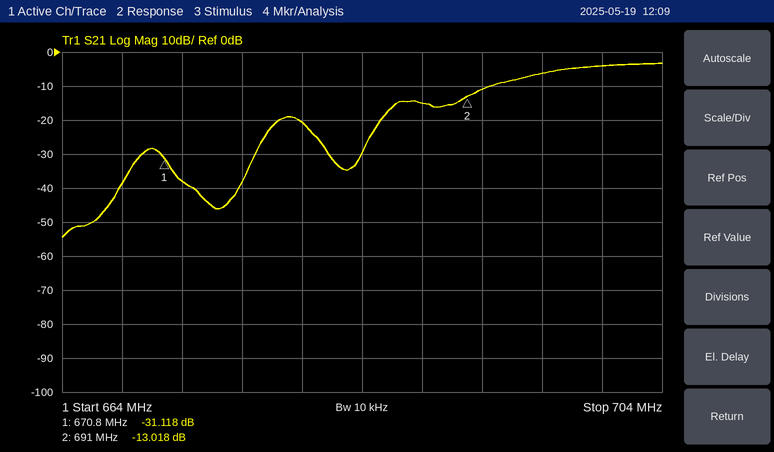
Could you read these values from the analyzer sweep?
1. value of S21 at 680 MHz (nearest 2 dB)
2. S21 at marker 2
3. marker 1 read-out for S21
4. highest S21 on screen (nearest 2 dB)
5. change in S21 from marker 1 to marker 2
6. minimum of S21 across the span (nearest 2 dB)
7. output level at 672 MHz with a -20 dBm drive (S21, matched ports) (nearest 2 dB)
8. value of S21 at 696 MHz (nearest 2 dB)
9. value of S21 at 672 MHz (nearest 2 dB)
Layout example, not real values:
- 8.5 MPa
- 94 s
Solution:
- -20 dB
- -13.018 dB
- -31.118 dB
- -4 dB
- 18.100 dB
- -54 dB
- -58 dBm
- -6 dB
- -38 dB
